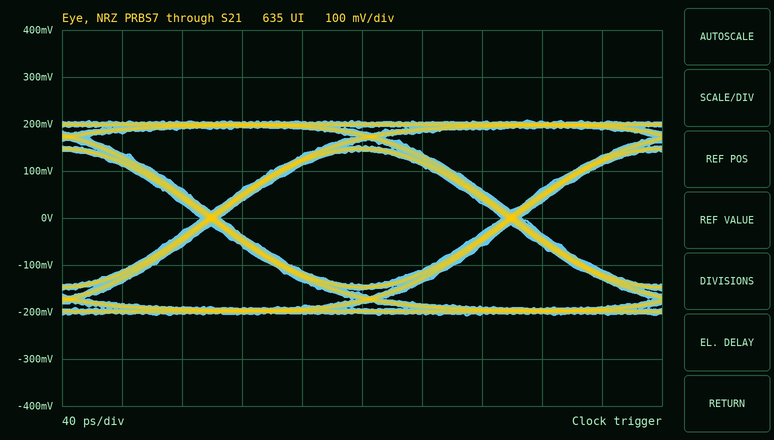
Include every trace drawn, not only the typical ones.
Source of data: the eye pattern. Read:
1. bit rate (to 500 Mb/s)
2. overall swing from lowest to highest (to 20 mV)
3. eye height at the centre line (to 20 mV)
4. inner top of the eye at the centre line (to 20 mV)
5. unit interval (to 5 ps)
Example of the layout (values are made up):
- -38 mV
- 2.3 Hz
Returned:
- 5.0 Gb/s
- 420 mV
- 280 mV
- 140 mV
- 200 ps
